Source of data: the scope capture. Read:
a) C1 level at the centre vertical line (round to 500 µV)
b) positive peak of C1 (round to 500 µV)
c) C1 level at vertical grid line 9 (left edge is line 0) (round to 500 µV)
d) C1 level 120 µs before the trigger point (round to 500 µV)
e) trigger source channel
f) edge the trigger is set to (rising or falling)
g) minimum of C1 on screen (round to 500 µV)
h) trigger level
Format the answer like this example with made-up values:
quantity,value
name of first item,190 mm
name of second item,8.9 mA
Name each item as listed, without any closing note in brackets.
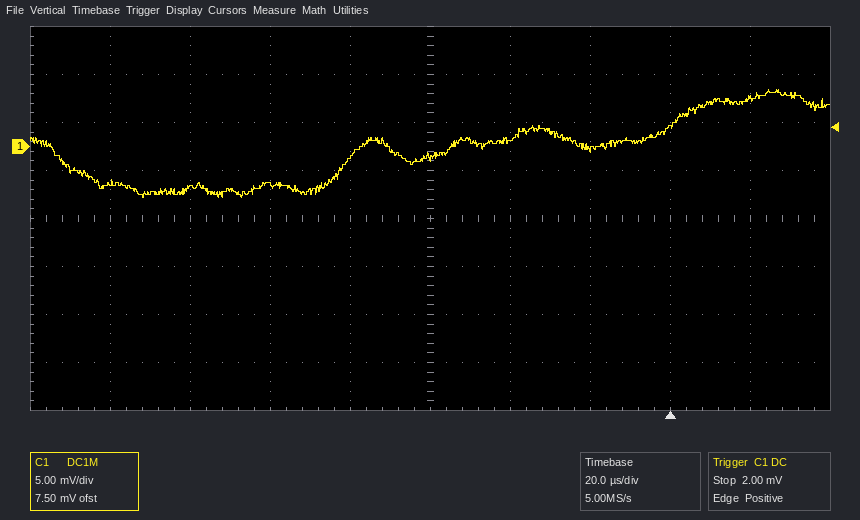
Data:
quantity,value
C1 level at the centre vertical line,-1.0 mV
positive peak of C1,6.0 mV
C1 level at vertical grid line 9 (left edge is line 0),5.0 mV
C1 level 120 µs before the trigger point,-4.5 mV
trigger source channel,C1
edge the trigger is set to,rising
minimum of C1 on screen,-5.5 mV
trigger level,2.00 mV
